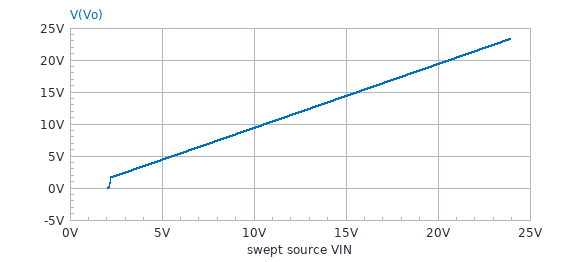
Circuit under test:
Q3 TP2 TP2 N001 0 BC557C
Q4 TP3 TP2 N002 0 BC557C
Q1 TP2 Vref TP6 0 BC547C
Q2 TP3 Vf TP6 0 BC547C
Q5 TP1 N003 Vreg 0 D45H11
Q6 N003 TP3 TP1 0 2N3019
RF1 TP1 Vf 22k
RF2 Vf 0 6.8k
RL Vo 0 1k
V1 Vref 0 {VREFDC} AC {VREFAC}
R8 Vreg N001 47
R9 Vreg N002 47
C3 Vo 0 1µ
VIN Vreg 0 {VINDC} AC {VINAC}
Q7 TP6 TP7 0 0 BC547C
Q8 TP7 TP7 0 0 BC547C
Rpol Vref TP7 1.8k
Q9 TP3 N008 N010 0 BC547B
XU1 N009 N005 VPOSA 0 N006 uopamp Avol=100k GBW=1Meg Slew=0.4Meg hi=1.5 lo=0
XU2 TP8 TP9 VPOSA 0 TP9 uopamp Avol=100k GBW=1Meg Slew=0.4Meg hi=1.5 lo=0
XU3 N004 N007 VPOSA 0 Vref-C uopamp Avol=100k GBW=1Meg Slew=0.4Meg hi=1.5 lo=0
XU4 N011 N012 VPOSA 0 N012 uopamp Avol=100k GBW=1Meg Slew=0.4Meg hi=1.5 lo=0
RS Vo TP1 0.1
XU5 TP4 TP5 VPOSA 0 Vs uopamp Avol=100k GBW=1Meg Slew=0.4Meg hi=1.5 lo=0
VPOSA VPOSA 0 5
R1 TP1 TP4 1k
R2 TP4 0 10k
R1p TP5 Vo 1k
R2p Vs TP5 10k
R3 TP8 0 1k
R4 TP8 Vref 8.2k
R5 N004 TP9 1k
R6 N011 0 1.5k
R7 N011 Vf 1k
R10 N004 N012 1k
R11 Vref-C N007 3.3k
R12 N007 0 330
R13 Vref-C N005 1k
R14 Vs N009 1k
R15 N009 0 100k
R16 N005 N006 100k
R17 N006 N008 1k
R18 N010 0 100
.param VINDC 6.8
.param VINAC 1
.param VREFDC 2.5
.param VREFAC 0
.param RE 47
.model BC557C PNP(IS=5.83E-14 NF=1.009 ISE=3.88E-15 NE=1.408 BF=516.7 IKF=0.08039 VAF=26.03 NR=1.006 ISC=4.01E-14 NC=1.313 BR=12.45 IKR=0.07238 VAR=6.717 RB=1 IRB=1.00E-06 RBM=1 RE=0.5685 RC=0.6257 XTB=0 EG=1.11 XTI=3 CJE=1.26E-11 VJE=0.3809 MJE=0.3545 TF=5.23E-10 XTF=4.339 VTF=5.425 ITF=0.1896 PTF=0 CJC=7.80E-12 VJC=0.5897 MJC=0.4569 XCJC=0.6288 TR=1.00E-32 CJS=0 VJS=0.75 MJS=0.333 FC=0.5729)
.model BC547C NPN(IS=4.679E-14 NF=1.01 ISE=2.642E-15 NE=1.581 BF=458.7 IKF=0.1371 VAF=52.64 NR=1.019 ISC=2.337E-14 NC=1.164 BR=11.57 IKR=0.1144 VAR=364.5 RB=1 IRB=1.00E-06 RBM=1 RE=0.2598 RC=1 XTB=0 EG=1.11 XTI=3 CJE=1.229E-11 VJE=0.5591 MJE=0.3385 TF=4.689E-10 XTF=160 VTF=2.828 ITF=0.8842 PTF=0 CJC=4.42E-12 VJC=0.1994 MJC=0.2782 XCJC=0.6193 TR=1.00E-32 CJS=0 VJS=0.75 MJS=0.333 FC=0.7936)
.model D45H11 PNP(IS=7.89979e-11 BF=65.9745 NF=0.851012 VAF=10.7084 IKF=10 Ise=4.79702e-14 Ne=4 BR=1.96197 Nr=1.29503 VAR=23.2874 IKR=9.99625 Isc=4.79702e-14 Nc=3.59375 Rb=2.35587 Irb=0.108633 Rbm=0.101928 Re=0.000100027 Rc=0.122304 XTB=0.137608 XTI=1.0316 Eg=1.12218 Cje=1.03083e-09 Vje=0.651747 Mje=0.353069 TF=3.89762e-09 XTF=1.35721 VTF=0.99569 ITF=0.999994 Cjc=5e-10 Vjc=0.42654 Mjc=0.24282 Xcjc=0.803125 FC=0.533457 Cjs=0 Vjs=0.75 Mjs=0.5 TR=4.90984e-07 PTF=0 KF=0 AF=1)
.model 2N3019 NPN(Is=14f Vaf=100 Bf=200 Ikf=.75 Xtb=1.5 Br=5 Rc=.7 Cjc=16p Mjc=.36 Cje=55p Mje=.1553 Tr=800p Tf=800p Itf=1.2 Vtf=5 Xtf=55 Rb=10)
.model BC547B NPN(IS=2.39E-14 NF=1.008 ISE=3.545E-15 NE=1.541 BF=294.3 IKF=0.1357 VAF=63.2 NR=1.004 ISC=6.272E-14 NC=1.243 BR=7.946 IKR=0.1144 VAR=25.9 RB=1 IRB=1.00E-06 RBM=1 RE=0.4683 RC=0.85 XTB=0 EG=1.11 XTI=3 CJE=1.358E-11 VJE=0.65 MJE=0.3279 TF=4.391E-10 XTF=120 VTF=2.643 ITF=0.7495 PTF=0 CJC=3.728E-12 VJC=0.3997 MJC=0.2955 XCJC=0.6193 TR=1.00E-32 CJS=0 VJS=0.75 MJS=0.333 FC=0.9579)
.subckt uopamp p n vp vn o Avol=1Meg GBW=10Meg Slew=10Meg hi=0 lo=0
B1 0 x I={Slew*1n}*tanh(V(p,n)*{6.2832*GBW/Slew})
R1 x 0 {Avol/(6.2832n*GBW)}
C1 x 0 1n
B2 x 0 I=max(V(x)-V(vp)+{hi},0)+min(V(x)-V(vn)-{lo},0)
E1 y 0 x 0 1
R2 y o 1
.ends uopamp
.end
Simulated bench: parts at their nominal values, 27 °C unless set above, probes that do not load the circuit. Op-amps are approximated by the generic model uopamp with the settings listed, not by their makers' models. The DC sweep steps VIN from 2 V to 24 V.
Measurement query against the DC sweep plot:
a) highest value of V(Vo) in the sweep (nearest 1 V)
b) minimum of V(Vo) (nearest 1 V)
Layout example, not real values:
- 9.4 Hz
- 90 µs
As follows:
- 23 V
- 0 V
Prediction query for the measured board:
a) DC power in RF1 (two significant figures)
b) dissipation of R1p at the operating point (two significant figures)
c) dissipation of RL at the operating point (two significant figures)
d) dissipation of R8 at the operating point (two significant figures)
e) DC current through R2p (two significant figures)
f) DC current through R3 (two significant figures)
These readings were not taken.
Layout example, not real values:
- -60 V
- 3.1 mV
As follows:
- 1.5 mW
- 320 µW
- 38 mW
- 33 µW
- 560 µA
- 270 µA
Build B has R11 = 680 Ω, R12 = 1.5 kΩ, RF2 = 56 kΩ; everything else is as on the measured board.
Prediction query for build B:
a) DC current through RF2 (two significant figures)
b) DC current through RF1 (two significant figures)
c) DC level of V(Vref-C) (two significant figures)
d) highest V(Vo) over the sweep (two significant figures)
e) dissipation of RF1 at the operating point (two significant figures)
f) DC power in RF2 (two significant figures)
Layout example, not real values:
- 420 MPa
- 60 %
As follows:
- 11 µA
- 250 µA
- 460 mV
- 23 V
- 1.4 mW
- 6.6 µW
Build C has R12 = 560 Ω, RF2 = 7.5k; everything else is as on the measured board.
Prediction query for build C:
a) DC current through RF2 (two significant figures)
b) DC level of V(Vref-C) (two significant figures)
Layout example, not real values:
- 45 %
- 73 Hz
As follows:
- 65 µA
- 1.9 V
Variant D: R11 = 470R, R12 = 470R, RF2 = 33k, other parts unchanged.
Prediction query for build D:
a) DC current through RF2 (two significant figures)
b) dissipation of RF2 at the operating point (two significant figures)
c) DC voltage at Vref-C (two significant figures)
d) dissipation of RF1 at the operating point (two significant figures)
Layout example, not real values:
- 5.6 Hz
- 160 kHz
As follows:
- 18 µA
- 11 µW
- 630 mV
- 1.4 mW
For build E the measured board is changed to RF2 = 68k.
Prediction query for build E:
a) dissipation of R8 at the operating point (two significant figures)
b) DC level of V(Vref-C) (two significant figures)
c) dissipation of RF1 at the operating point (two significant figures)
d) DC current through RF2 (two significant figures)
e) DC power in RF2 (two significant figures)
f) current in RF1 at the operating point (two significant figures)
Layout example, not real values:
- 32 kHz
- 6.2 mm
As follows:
- 33 µW
- 3.5 V
- 1.4 mW
- 9.0 µA
- 5.5 µW
- 250 µA
